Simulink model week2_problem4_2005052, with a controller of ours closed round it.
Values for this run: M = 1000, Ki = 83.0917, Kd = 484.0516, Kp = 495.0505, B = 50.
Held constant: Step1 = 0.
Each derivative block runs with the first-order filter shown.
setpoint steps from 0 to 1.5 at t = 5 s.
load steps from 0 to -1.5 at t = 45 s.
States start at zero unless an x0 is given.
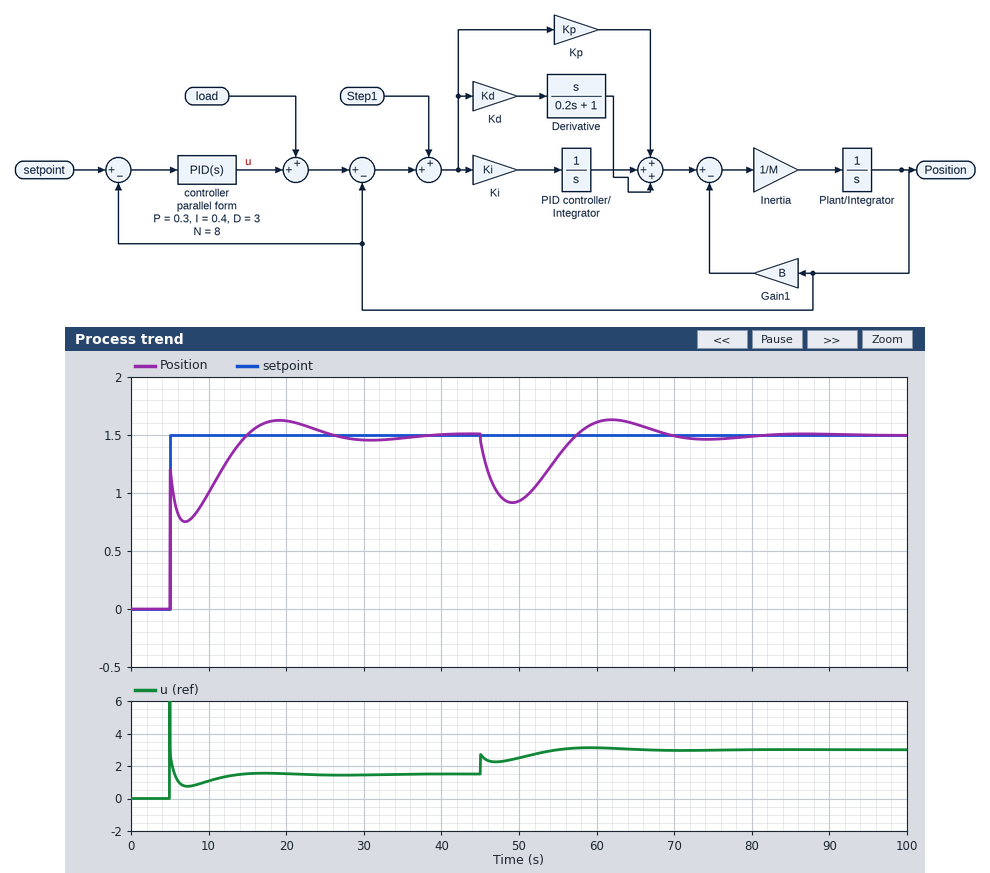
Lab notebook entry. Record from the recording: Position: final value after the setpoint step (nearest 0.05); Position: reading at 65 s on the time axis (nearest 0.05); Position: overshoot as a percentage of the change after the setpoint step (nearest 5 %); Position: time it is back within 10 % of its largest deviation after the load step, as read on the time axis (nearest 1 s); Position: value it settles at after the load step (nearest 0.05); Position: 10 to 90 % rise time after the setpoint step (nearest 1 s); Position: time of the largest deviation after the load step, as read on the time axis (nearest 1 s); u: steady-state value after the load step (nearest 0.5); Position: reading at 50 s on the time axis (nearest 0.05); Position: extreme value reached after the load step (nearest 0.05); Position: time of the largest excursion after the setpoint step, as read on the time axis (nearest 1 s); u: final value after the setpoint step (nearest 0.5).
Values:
1.50
1.60
10 %
67 s
1.50
8 s
49 s
3.0
0.95
0.90
19 s
1.5
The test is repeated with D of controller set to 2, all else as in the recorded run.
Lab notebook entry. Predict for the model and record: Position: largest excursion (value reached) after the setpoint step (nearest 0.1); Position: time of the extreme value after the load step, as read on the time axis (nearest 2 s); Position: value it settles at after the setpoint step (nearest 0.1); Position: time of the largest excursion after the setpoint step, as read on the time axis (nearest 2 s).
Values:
1.6
48 s
1.5
18 s
